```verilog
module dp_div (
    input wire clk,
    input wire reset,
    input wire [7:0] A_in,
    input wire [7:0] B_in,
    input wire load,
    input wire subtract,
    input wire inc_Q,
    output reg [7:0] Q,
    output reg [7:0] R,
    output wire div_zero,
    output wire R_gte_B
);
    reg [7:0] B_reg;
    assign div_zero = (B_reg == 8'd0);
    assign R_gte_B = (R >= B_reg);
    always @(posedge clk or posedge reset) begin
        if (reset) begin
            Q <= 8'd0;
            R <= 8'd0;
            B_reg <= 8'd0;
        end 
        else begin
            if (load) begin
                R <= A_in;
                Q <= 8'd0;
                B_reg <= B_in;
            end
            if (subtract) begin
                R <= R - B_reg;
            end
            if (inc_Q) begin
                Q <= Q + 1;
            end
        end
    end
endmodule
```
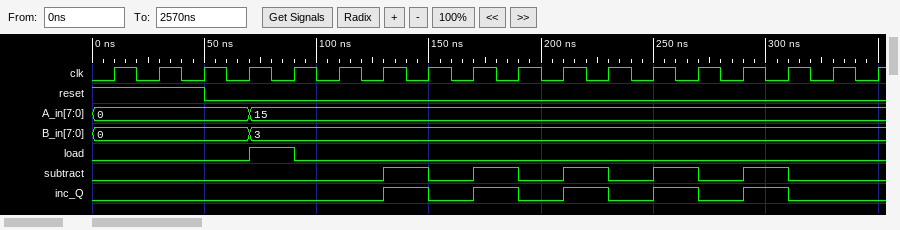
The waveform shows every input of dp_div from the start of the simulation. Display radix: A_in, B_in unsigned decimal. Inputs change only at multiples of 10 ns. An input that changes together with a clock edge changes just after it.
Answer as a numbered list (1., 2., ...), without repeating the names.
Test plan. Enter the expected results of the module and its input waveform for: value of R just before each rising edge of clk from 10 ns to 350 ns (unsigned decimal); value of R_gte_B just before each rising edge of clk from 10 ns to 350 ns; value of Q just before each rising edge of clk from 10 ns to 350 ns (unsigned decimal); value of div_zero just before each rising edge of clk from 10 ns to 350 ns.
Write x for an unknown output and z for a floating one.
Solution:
1. 0, 0, 0, 0, 0, 15, 15, 15, 12, 12, 9, 9, 6, 6, 3, 3, 0, 0
2. 1 1 1 1 1 1 1 1 1 1 1 1 1 1 1 1 0 0
3. 0, 0, 0, 0, 0, 0, 0, 0, 1, 1, 2, 2, 3, 3, 4, 4, 5, 5
4. 1 1 1 1 1 0 0 0 0 0 0 0 0 0 0 0 0 0
